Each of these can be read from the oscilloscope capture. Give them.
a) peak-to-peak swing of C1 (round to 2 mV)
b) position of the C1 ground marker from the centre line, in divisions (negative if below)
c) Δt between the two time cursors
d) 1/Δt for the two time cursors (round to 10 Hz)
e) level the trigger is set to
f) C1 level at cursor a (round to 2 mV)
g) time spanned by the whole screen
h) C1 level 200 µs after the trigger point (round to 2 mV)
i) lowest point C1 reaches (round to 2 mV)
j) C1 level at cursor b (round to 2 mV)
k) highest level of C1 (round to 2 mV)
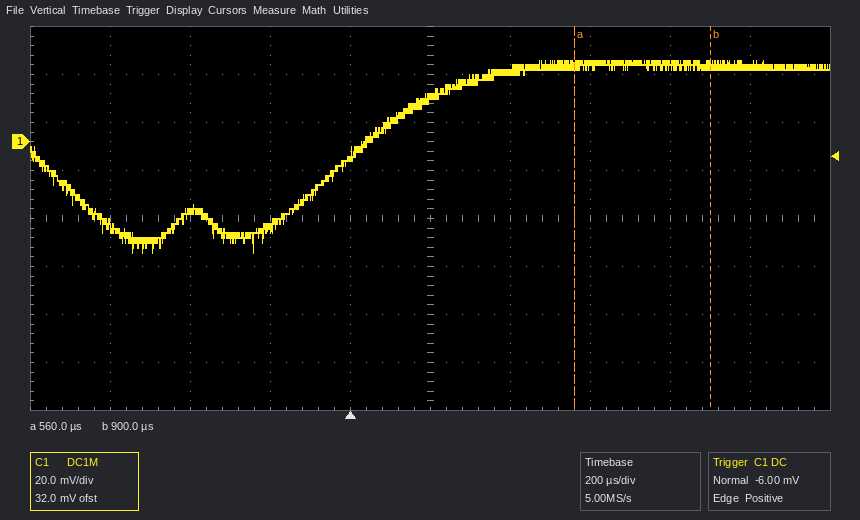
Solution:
80 mV
+1.6 div
340 µs
2.94 kHz
-6.00 mV
32 mV
2 ms
18 mV
-46 mV
32 mV
34 mV
